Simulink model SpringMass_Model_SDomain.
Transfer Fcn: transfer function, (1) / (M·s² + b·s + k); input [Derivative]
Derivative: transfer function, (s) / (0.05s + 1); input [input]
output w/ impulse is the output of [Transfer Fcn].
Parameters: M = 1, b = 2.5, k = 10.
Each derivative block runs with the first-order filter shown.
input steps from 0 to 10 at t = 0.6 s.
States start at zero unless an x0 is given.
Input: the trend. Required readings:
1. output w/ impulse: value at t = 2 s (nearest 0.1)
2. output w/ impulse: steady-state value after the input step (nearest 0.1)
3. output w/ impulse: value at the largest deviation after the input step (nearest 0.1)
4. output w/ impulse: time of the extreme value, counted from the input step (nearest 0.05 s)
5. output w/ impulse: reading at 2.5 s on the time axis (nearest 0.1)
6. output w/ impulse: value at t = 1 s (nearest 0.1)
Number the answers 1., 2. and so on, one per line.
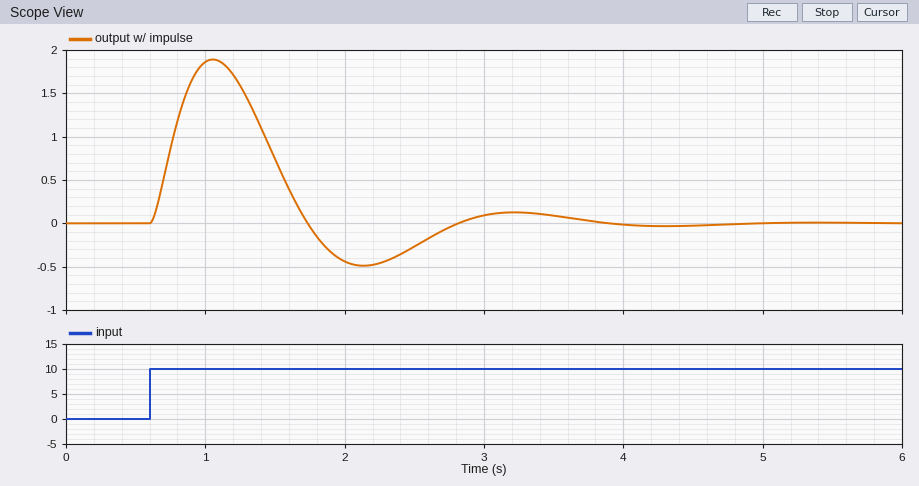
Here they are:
1. -0.4
2. 0.0
3. 1.9
4. 0.45 s
5. -0.3
6. 1.9
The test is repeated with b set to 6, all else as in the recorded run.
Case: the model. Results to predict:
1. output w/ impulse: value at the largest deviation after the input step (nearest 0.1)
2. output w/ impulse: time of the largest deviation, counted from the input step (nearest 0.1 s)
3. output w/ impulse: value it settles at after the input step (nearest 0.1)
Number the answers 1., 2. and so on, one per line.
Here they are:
1. 1.2
2. 0.4 s
3. 0.0
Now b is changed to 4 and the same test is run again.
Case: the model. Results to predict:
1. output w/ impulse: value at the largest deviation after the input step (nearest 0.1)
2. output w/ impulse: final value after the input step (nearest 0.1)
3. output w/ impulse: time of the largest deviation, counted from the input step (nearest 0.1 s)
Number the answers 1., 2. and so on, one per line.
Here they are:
1. 1.5
2. 0.0
3. 0.4 s
